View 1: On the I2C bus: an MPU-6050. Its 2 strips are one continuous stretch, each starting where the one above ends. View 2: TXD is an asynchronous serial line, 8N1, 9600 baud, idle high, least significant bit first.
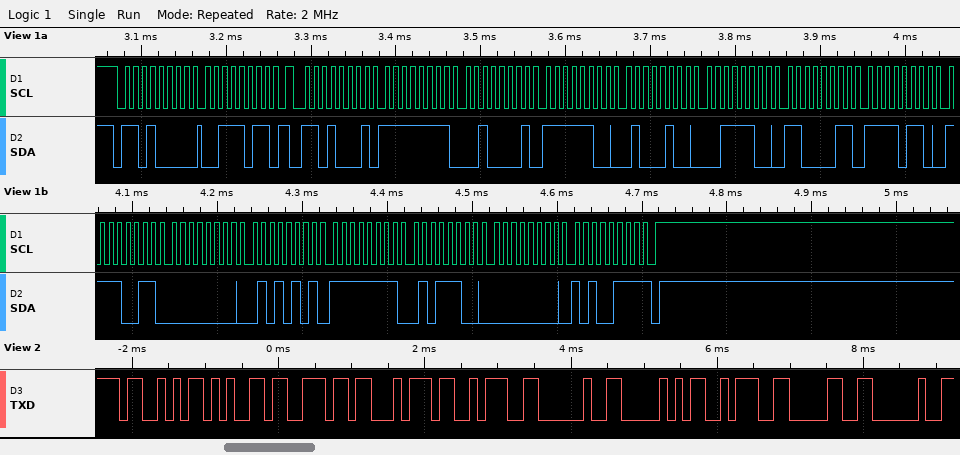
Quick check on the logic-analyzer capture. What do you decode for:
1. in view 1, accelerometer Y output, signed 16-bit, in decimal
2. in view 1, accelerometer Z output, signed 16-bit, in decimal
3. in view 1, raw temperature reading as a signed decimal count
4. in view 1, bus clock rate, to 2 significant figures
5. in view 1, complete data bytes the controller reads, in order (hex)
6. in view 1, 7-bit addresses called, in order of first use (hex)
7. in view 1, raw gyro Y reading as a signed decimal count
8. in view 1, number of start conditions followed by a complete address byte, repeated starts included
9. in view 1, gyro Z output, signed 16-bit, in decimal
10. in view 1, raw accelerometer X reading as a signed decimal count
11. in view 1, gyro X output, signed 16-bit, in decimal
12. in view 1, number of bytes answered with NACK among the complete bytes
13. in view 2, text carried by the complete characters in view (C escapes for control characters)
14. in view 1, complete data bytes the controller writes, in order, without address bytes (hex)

-956
15555
-2317
100 kHz
FF 21 FC 44 3C C3 F6 F3 00 55 FF 5C 00 A7
0x68
-164
2
167
-223
85
1
"Sent: P:0 "
3B
